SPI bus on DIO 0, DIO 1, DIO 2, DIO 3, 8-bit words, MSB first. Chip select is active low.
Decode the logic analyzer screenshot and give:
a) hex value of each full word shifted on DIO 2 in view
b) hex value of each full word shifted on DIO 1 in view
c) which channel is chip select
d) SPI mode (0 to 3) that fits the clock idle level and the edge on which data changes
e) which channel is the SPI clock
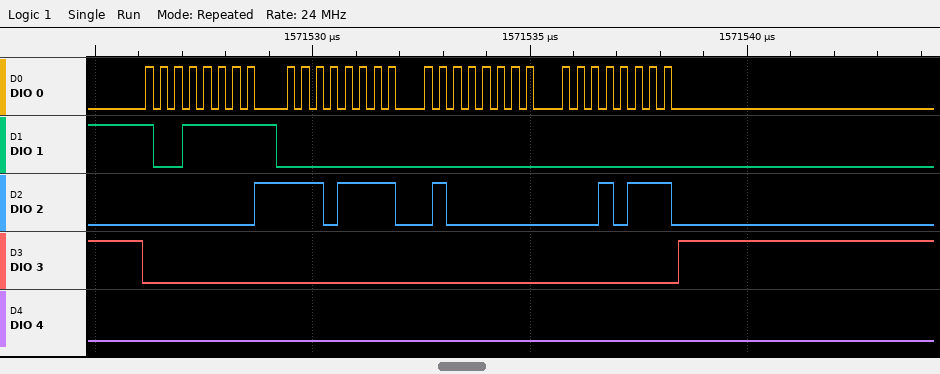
00, EF, 40, 17
9F, 00, 00, 00
DIO 3
0
DIO 0
